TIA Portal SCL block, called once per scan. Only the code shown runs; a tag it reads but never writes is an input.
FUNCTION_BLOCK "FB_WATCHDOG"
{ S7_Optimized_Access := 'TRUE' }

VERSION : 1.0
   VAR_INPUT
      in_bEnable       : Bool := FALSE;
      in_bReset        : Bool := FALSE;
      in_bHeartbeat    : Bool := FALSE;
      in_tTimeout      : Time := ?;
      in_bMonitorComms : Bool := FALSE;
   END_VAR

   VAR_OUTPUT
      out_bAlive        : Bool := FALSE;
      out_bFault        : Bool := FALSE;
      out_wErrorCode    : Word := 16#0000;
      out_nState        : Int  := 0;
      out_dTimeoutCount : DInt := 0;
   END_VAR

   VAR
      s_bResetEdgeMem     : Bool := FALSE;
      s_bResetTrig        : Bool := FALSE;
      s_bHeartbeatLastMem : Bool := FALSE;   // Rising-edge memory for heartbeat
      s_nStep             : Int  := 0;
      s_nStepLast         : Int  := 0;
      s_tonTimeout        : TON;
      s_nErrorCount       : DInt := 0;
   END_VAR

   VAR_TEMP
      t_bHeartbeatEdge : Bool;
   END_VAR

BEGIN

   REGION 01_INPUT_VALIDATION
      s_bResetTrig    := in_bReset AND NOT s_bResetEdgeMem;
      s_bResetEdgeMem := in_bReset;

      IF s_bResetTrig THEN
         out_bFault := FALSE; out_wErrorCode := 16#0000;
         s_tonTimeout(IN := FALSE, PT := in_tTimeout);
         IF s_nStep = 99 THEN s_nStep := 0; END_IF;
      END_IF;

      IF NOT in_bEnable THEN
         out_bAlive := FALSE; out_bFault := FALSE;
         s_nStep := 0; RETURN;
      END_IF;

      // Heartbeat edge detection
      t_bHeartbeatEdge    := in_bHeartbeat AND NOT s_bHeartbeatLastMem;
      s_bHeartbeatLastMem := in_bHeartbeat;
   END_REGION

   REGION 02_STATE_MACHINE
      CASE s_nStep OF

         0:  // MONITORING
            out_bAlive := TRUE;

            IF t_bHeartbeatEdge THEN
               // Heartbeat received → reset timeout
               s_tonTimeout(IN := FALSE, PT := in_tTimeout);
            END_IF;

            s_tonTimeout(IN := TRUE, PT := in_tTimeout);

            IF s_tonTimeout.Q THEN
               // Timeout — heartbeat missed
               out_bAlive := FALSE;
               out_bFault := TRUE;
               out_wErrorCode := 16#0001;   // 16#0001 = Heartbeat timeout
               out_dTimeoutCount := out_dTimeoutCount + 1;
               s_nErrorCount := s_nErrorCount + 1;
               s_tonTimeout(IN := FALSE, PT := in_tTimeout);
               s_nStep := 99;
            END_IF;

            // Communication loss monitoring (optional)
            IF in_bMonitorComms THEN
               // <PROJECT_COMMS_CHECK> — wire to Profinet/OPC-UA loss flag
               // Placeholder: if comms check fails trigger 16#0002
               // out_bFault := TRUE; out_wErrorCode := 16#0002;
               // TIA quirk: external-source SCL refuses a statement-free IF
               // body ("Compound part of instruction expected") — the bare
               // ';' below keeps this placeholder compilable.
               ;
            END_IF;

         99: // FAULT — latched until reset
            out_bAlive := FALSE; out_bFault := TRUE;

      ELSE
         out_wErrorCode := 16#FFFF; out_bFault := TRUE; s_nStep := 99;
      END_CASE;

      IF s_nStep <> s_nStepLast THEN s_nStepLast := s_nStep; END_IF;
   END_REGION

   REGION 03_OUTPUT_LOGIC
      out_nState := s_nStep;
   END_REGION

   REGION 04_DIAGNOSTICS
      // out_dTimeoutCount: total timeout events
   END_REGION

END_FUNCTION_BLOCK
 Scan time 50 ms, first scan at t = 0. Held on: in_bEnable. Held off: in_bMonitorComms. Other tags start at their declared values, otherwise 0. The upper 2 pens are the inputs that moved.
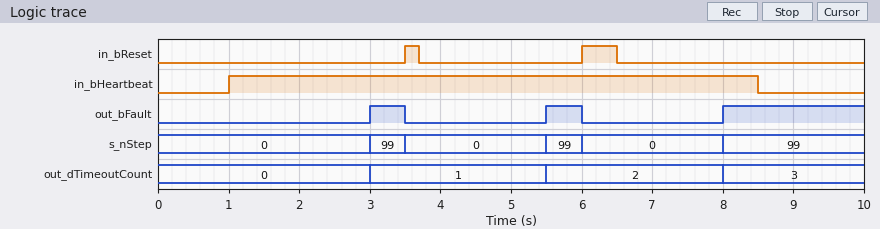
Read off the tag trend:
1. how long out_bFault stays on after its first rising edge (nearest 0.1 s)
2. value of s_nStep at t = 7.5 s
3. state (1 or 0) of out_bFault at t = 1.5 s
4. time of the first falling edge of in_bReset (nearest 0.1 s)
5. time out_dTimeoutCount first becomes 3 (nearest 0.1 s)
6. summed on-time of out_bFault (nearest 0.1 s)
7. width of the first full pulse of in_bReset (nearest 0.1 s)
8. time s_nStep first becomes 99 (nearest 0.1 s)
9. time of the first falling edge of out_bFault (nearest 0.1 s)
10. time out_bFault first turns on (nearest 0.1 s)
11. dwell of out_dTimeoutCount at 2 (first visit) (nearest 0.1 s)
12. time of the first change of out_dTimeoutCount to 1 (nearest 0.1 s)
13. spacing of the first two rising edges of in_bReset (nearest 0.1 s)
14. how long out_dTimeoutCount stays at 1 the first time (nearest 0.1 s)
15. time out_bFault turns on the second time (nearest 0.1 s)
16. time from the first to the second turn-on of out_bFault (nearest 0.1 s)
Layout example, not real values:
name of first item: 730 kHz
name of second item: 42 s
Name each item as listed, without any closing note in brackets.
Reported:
how long out_bFault stays on after its first rising edge: 0.5 s
value of s_nStep at t = 7.5 s: 0
state (1 or 0) of out_bFault at t = 1.5 s: 0
time of the first falling edge of in_bReset: 3.7 s
time out_dTimeoutCount first becomes 3: 8.0 s
summed on-time of out_bFault: 3.0 s
width of the first full pulse of in_bReset: 0.2 s
time s_nStep first becomes 99: 3.0 s
time of the first falling edge of out_bFault: 3.5 s
time out_bFault first turns on: 3.0 s
dwell of out_dTimeoutCount at 2 (first visit): 2.5 s
time of the first change of out_dTimeoutCount to 1: 3.0 s
spacing of the first two rising edges of in_bReset: 2.5 s
how long out_dTimeoutCount stays at 1 the first time: 2.5 s
time out_bFault turns on the second time: 5.5 s
time from the first to the second turn-on of out_bFault: 2.5 s
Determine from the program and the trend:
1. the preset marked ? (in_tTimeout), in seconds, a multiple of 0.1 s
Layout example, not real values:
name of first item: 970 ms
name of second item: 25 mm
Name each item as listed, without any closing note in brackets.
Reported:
the preset marked ? (in_tTimeout), in seconds, a multiple of 0.1 s: 2.0 s
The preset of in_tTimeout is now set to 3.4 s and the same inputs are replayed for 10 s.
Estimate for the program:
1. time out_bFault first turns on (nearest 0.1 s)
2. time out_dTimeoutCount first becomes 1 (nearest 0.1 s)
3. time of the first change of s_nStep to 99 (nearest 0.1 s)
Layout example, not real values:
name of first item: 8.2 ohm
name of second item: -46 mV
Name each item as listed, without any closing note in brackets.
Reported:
time out_bFault first turns on: 9.4 s
time out_dTimeoutCount first becomes 1: 9.4 s
time of the first change of s_nStep to 99: 9.4 s
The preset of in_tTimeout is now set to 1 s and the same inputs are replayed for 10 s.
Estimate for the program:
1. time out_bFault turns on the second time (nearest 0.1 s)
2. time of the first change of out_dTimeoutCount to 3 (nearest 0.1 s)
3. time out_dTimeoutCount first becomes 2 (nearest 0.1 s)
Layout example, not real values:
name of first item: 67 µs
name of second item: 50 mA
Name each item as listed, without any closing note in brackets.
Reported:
time out_bFault turns on the second time: 4.5 s
time of the first change of out_dTimeoutCount to 3: 7.0 s
time out_dTimeoutCount first becomes 2: 4.5 s
